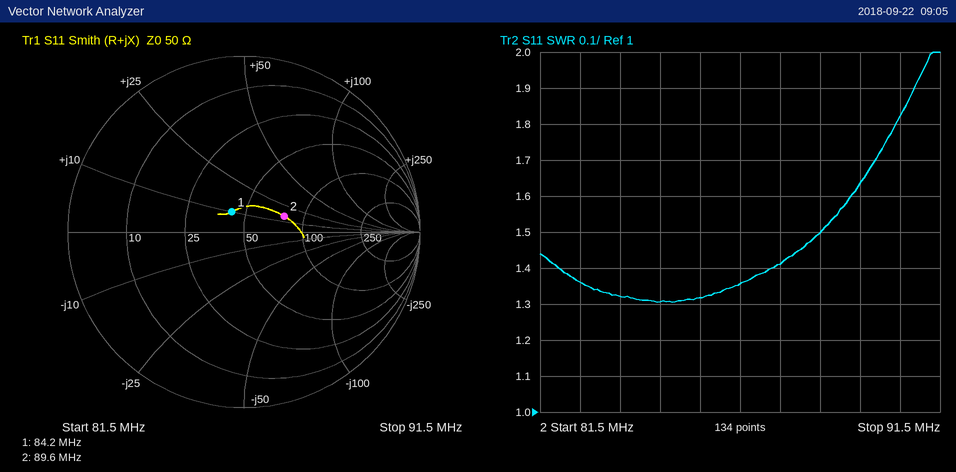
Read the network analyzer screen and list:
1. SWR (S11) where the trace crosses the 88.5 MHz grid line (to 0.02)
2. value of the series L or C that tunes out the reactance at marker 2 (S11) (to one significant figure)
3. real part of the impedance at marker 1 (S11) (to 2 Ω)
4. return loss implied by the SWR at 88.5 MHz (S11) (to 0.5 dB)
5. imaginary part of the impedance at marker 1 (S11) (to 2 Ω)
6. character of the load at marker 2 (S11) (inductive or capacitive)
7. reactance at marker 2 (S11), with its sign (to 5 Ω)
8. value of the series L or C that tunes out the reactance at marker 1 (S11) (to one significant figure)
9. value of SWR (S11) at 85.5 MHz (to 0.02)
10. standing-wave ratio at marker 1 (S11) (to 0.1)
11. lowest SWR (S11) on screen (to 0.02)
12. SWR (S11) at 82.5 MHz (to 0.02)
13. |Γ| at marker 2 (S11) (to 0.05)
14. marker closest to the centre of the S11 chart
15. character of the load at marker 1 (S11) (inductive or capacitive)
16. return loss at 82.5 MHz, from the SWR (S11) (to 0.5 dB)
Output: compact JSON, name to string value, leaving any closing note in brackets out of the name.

{"SWR (S11) where the trace crosses the 88.5 MHz grid line": "1.50", "value of the series L or C that tunes out the reactance at marker 2 (S11)": "100 pF", "real part of the impedance at marker 1 (S11)": "42 Ω", "return loss implied by the SWR at 88.5 MHz (S11)": "14.0 dB", "imaginary part of the impedance at marker 1 (S11)": "+10 Ω", "character of the load at marker 2 (S11)": "inductive", "reactance at marker 2 (S11), with its sign": "+15 Ω", "value of the series L or C that tunes out the reactance at marker 1 (S11)": "200 pF", "value of SWR (S11) at 85.5 MHz": "1.32", "standing-wave ratio at marker 1 (S11)": "1.3", "lowest SWR (S11) on screen": "1.30", "SWR (S11) at 82.5 MHz": "1.36", "|Γ| at marker 2 (S11)": "0.25", "marker closest to the centre of the S11 chart": "marker 1", "character of the load at marker 1 (S11)": "inductive", "return loss at 82.5 MHz, from the SWR (S11)": "16.5 dB"}
